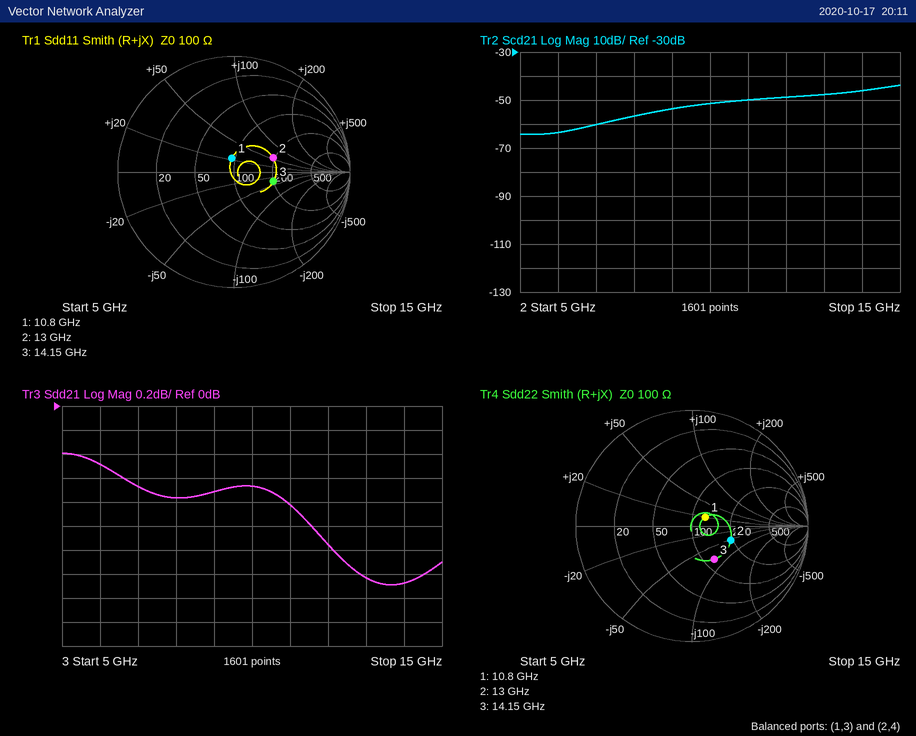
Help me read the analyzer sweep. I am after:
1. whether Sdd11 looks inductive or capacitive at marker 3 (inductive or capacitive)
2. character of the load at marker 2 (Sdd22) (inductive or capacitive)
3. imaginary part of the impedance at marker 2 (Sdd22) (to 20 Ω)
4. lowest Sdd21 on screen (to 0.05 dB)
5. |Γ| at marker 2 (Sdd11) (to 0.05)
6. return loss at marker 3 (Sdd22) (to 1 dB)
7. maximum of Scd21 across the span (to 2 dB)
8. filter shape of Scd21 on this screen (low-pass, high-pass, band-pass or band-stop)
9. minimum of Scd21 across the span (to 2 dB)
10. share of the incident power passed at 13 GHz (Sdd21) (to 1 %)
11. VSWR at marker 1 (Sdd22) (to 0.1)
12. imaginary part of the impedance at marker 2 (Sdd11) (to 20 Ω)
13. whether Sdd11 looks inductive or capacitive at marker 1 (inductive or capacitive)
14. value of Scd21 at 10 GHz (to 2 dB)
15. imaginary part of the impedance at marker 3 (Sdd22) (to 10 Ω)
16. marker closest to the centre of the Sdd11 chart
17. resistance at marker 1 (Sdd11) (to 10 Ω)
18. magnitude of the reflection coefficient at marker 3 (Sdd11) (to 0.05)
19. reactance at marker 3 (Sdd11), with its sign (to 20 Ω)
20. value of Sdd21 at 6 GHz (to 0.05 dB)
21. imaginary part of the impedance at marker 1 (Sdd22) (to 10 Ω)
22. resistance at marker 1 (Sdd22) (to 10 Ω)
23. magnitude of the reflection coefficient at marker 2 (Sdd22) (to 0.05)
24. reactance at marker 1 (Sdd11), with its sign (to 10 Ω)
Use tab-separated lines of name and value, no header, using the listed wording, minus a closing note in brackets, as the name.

whether Sdd11 looks inductive or capacitive at marker 3	capacitive
character of the load at marker 2 (Sdd22)	capacitive
imaginary part of the impedance at marker 2 (Sdd22)	-60 Ω
lowest Sdd21 on screen	-1.50 dB
|Γ| at marker 2 (Sdd11)	0.35
return loss at marker 3 (Sdd22)	9 dB
maximum of Scd21 across the span	-44 dB
filter shape of Scd21 on this screen	high-pass
minimum of Scd21 across the span	-64 dB
share of the incident power passed at 13 GHz (Sdd21)	72 %
VSWR at marker 1 (Sdd22)	1.3
imaginary part of the impedance at marker 2 (Sdd11)	+60 Ω
whether Sdd11 looks inductive or capacitive at marker 1	inductive
value of Scd21 at 10 GHz	-52 dB
imaginary part of the impedance at marker 3 (Sdd22)	-80 Ω
marker closest to the centre of the Sdd11 chart	marker 1
resistance at marker 1 (Sdd11)	90 Ω
magnitude of the reflection coefficient at marker 3 (Sdd11)	0.35
reactance at marker 3 (Sdd11), with its sign	-40 Ω
value of Sdd21 at 6 GHz	-0.50 dB
imaginary part of the impedance at marker 1 (Sdd22)	+20 Ω
resistance at marker 1 (Sdd22)	120 Ω
magnitude of the reflection coefficient at marker 2 (Sdd22)	0.35
reactance at marker 1 (Sdd11), with its sign	+20 Ω
